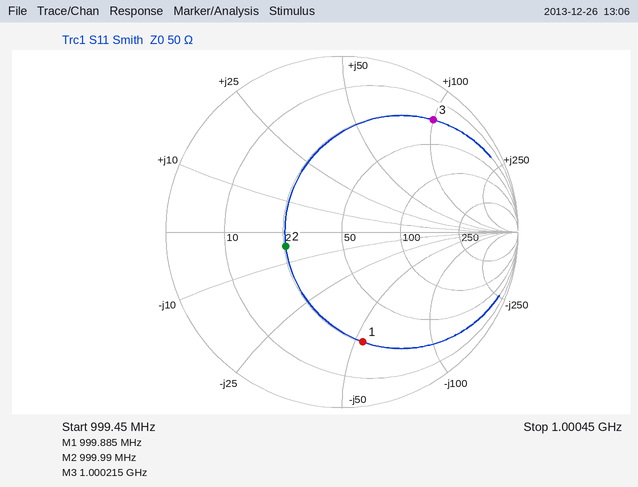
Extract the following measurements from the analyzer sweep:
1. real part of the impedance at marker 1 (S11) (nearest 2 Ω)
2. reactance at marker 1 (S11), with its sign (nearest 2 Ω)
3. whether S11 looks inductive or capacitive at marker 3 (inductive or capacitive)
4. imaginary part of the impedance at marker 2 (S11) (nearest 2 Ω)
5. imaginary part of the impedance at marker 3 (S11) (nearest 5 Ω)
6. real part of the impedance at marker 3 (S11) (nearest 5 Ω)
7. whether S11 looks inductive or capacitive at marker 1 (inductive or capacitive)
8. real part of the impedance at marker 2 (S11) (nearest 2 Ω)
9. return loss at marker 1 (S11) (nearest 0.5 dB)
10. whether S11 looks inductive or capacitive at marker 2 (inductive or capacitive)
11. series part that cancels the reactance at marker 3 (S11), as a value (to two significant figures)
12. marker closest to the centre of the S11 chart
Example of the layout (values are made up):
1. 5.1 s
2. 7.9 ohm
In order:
1. 26 Ω
2. -54 Ω
3. inductive
4. -4 Ω
5. +100 Ω
6. 25 Ω
7. capacitive
8. 26 Ω
9. 4.0 dB
10. capacitive
11. 1.6 pF
12. marker 2
